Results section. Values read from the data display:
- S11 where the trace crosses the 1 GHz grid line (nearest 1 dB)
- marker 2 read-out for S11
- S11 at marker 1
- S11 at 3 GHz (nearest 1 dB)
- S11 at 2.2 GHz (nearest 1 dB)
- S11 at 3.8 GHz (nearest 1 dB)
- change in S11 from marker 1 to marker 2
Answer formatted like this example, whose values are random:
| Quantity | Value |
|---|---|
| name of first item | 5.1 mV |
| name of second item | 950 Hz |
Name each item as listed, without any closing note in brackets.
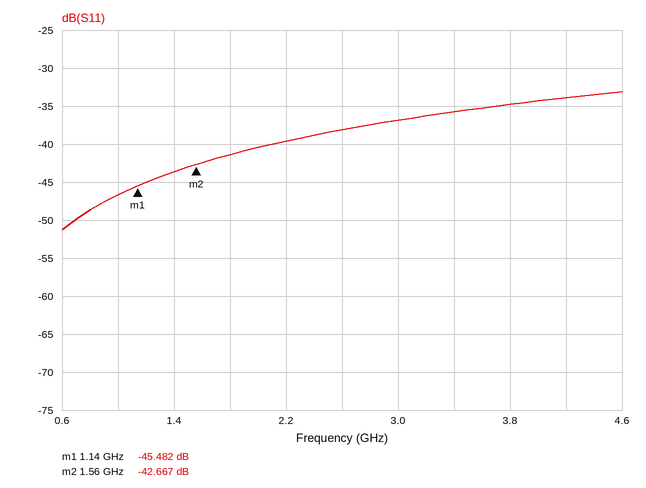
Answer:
| Quantity | Value |
|---|---|
| S11 where the trace crosses the 1 GHz grid line | -47 dB |
| marker 2 read-out for S11 | -42.667 dB |
| S11 at marker 1 | -45.482 dB |
| S11 at 3 GHz | -37 dB |
| S11 at 2.2 GHz | -40 dB |
| S11 at 3.8 GHz | -35 dB |
| change in S11 from marker 1 to marker 2 | 2.815 dB |
